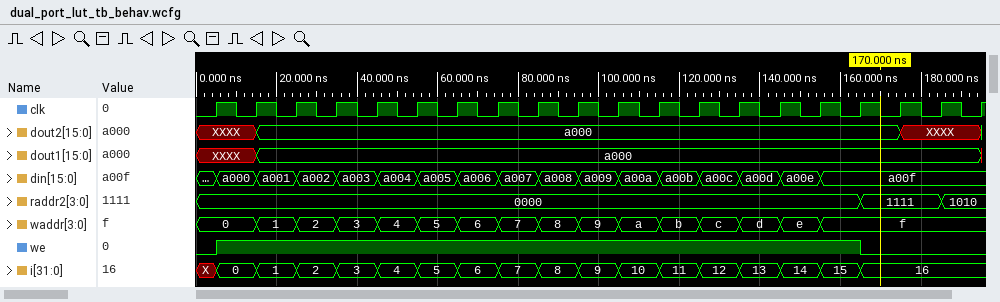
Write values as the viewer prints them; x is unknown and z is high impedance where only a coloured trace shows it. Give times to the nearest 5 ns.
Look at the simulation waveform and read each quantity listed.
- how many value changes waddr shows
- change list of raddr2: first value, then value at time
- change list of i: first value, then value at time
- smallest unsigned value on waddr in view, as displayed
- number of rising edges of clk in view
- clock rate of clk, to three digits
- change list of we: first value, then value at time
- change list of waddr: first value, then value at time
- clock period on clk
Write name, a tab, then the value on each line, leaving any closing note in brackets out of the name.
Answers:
how many value changes waddr shows	15
change list of raddr2: first value, then value at time	0000, 1111 at 165 ns, 1010 at 185 ns
change list of i: first value, then value at time	X, 0 at 5 ns, 1 at 15 ns, 2 at 25 ns, 3 at 35 ns, 4 at 45 ns, 5 at 55 ns, 6 at 65 ns, 7 at 75 ns, 8 at 85 ns, 9 at 95 ns, 10 at 105 ns, 11 at 115 ns, 12 at 125 ns, 13 at 135 ns, 14 at 145 ns, 15 at 155 ns, 16 at 165 ns
smallest unsigned value on waddr in view, as displayed	0
number of rising edges of clk in view	20
clock rate of clk, to three digits	100 MHz
change list of we: first value, then value at time	0, 1 at 5 ns, 0 at 165 ns
change list of waddr: first value, then value at time	0, 1 at 15 ns, 2 at 25 ns, 3 at 35 ns, 4 at 45 ns, 5 at 55 ns, 6 at 65 ns, 7 at 75 ns, 8 at 85 ns, 9 at 95 ns, a at 105 ns, b at 115 ns, c at 125 ns, d at 135 ns, e at 145 ns, f at 155 ns
clock period on clk	10 ns
